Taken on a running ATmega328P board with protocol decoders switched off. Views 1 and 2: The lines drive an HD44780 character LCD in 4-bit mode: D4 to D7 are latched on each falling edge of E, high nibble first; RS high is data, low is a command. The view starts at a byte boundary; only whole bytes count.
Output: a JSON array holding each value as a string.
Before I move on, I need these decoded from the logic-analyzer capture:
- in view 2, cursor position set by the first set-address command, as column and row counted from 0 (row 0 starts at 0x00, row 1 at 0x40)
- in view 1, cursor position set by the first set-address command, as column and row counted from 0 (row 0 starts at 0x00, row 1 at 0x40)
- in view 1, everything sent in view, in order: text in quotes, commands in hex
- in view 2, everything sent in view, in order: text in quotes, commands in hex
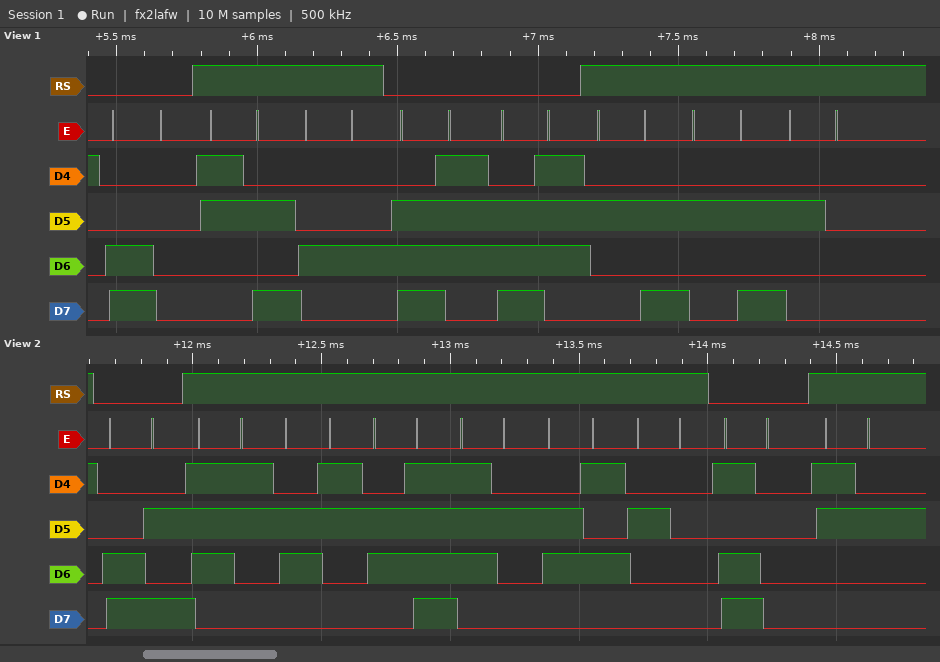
["column 10, row 1", "column 0, row 1", "0xC0 \":D\" 0xE7 0xE7 \"** \"", "0xCA \"score \" 0xD0 \"2\""]
